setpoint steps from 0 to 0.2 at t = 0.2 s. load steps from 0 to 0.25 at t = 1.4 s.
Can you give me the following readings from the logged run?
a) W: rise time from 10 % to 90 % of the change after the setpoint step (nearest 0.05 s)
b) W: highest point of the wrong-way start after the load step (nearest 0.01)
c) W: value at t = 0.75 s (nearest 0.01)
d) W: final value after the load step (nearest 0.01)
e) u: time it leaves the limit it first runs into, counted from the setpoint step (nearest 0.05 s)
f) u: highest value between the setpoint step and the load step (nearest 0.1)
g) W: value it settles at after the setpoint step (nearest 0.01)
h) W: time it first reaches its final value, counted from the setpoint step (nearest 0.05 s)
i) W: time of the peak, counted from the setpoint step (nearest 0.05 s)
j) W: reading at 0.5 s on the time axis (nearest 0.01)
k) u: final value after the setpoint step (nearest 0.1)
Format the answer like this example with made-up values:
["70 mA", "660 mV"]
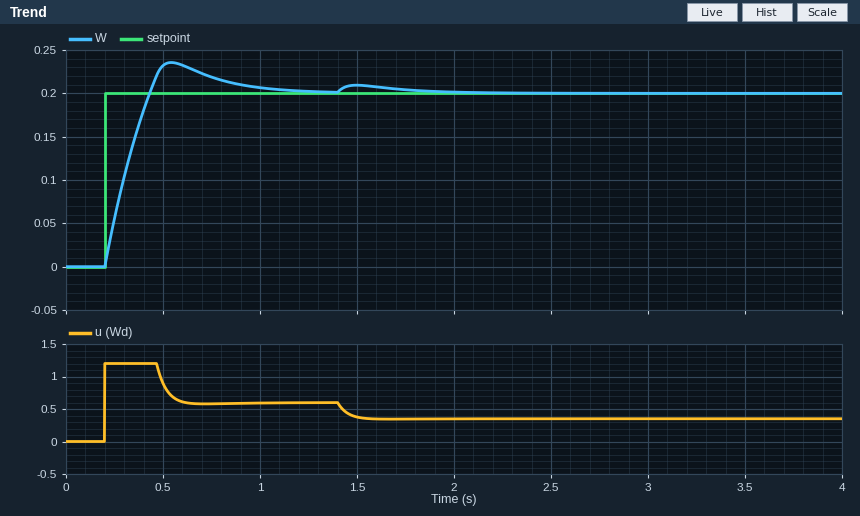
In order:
["0.20 s", "0.21", "0.22", "0.20", "0.25 s", "1.2", "0.20", "0.25 s", "0.35 s", "0.23", "0.6"]
